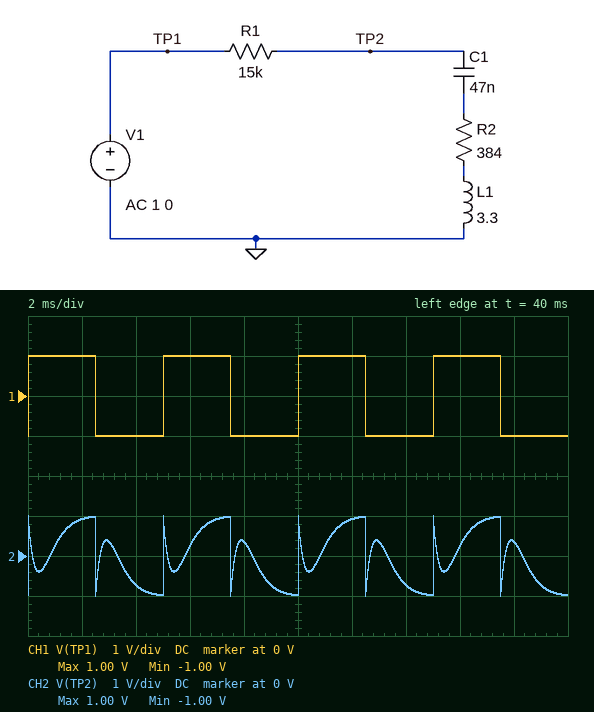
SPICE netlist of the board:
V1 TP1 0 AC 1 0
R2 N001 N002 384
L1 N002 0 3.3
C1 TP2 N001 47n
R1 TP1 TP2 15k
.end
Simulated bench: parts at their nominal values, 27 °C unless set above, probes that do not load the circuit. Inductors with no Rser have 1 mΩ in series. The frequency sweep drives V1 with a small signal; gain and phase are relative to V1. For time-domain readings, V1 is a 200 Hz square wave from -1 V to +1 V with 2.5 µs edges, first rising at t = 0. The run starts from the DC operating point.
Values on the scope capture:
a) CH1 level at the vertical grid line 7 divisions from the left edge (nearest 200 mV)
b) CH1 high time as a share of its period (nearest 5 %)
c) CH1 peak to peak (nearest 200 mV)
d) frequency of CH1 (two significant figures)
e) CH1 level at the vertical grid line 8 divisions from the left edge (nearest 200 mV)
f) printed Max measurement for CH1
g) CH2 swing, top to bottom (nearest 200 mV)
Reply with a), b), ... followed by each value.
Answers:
a) -1.0 V
b) 50 %
c) 2.0 V
d) 200 Hz
e) 1.0 V
f) 1.00 V
g) 2.0 V
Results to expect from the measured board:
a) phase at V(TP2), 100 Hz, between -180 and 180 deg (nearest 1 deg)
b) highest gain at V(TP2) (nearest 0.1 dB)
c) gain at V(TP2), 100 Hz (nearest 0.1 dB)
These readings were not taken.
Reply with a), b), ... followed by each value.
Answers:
a) -25 deg
b) 0 dB
c) -0.9 dB
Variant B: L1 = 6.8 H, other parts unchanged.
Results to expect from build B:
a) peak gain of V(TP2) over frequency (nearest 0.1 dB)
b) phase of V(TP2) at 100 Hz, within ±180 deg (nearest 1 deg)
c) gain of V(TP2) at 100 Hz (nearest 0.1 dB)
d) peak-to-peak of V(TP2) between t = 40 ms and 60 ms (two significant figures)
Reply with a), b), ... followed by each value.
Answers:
a) 0 dB
b) -27 deg
c) -1.0 dB
d) 2.1 V
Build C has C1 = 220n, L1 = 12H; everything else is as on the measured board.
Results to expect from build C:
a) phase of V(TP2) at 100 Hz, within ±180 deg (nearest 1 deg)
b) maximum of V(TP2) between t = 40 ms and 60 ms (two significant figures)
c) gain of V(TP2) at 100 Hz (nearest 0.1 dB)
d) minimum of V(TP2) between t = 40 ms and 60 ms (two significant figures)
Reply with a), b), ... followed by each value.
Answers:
a) 37 deg
b) 1.9 V
c) -29.9 dB
d) -1.9 V
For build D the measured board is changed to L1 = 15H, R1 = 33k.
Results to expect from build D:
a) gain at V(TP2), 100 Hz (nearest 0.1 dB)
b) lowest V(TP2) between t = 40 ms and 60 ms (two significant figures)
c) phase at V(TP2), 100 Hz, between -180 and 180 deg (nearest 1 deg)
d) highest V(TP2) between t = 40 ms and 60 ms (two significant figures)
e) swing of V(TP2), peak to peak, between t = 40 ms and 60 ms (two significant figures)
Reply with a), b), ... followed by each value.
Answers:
a) -4.6 dB
b) -1.5 V
c) -53 deg
d) 1.5 V
e) 3.0 V
